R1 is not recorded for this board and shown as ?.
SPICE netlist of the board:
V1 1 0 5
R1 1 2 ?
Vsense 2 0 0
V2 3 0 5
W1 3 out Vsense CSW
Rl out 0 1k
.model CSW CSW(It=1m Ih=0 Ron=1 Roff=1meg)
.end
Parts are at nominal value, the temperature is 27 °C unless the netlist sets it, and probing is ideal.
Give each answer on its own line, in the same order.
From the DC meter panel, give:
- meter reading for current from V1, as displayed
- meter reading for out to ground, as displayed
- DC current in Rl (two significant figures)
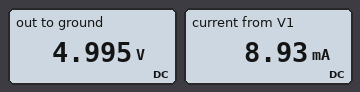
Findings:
8.93 mA
4.995 V
5.0 mA
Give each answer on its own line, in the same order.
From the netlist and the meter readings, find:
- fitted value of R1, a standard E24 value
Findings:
560 Ω
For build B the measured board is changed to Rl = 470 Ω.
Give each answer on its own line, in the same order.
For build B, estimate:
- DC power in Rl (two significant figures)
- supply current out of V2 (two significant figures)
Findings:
53 mW
11 mA
